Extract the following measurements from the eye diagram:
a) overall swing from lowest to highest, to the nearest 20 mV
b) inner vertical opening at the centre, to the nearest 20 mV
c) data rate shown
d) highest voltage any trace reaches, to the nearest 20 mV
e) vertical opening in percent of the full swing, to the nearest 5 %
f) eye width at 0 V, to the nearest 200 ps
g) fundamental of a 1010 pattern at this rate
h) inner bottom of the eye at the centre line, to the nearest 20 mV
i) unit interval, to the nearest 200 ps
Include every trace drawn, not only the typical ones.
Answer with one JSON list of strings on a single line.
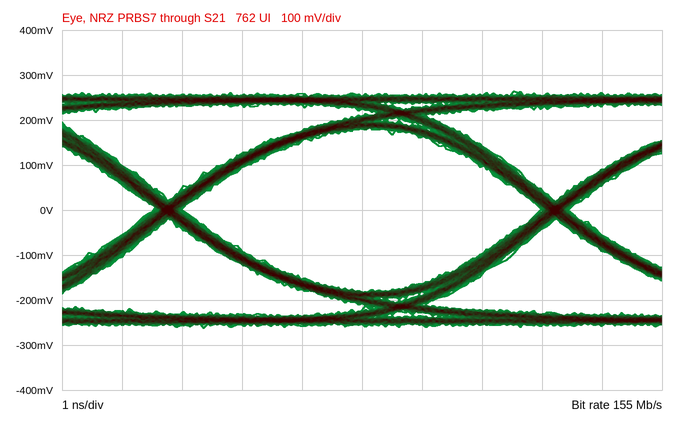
["520 mV", "360 mV", "155 Mb/s", "260 mV", "70 %", "6.0 ns", "77.5 MHz", "-180 mV", "6.4 ns"]
